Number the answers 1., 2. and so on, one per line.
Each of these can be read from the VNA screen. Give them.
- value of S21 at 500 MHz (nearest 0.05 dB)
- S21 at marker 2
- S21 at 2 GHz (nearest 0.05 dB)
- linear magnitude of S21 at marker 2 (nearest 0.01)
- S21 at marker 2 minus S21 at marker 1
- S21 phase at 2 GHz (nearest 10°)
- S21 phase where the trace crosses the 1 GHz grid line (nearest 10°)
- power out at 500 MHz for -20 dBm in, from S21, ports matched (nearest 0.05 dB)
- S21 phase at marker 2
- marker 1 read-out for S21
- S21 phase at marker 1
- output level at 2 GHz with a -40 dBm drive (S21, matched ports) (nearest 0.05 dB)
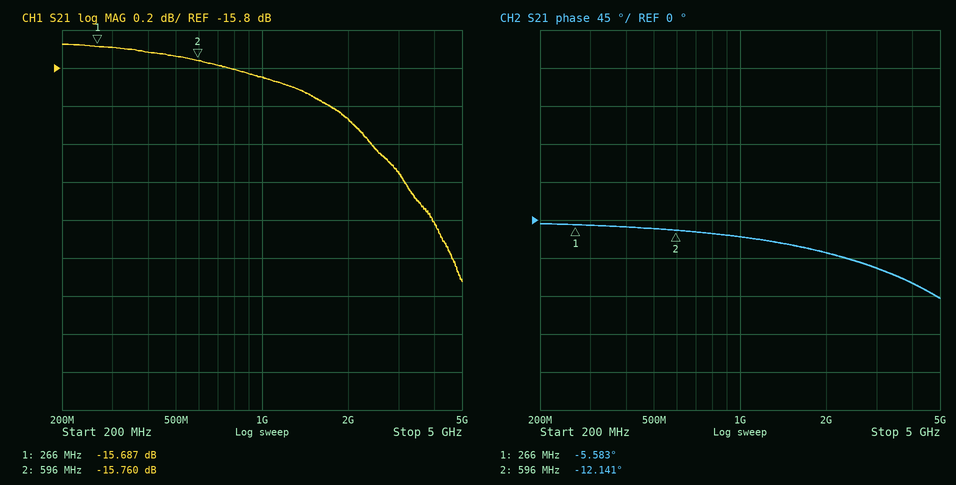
1. -15.75 dB
2. -15.760 dB
3. -16.05 dB
4. 0.16
5. -0.073 dB
6. -40°
7. -20°
8. -35.75 dBm
9. -12.141°
10. -15.687 dB
11. -5.583°
12. -56.05 dBm
